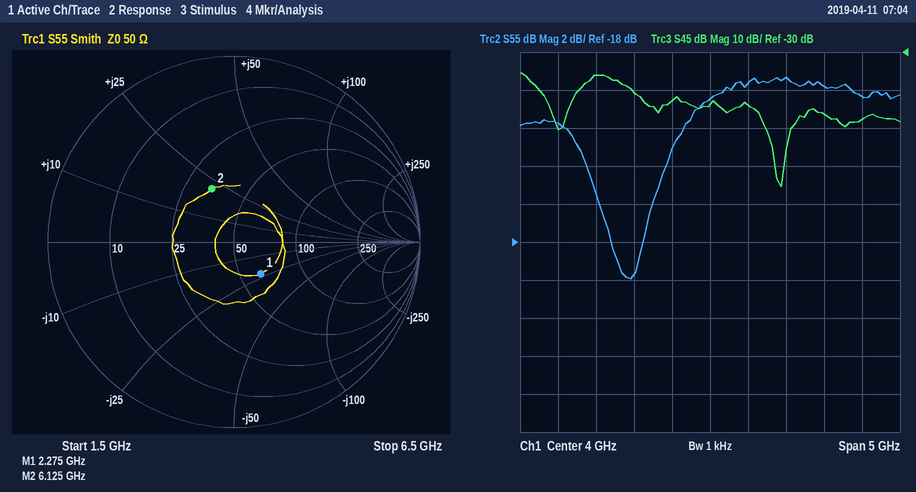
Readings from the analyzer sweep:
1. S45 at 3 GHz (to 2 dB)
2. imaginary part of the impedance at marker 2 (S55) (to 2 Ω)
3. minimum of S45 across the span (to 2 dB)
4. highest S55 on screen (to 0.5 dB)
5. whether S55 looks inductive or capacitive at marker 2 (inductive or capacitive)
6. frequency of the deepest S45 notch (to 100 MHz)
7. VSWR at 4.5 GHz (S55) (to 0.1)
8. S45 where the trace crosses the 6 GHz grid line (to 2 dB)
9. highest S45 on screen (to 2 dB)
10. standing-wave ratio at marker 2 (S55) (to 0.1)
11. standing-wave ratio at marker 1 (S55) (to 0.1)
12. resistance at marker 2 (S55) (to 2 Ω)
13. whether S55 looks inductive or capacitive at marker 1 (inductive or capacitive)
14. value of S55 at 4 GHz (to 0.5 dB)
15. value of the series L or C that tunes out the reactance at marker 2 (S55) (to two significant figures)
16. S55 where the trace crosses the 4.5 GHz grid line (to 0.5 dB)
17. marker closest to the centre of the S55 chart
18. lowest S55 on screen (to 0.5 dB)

-40 dB
+22 Ω
-66 dB
-9.5 dB
inductive
4.9 GHz
2.0
-48 dB
-36 dB
1.9
1.6
34 Ω
capacitive
-10.5 dB
1.2 pF
-9.5 dB
marker 1
-20.0 dB
